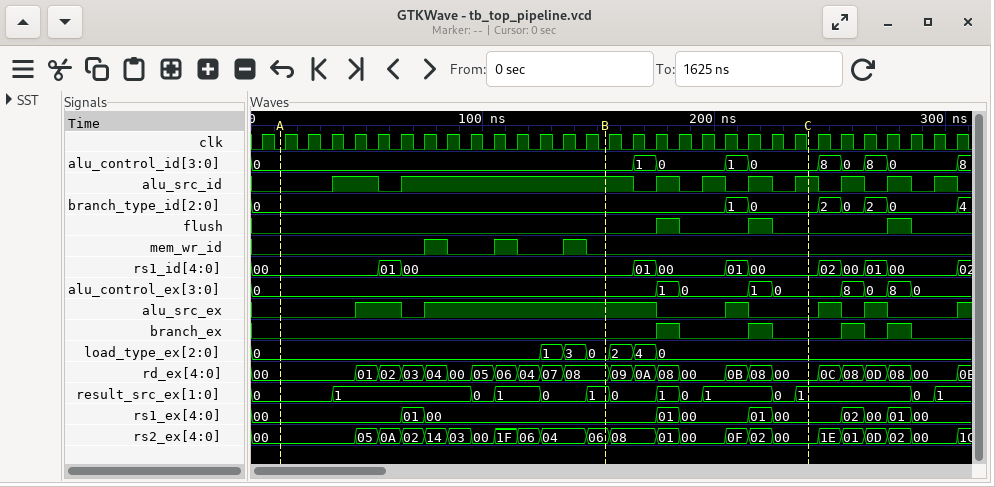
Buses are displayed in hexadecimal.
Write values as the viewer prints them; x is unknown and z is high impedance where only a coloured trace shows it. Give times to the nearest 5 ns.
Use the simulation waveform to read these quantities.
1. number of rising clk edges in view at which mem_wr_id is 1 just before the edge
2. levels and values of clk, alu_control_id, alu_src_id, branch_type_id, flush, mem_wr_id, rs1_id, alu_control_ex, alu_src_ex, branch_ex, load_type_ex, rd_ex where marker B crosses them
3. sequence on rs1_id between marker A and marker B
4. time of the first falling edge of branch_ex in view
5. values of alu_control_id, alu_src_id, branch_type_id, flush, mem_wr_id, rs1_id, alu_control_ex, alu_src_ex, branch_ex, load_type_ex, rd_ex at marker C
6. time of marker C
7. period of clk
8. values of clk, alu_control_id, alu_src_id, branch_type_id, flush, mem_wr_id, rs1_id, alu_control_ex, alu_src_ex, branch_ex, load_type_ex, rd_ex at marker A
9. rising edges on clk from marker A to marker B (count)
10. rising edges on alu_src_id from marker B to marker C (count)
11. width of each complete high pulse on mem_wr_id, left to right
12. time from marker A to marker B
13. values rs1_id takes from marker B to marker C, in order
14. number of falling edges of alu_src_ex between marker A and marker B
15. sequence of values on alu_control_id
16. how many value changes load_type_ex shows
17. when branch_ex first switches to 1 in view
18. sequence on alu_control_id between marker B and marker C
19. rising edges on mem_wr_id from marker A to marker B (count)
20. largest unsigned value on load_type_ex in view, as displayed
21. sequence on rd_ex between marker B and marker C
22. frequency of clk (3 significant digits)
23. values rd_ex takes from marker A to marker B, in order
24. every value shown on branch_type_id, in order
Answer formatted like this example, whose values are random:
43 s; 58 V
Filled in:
3; clk=0, alu_control_id=0, alu_src_id=1, branch_type_id=0, flush=0, mem_wr_id=0, rs1_id=00, alu_control_ex=0, alu_src_ex=1, branch_ex=0, load_type_ex=0, rd_ex=08; 00, 01, 00; 185 ns; alu_control_id=0, alu_src_id=1, branch_type_id=0, flush=0, mem_wr_id=0, rs1_id=00, alu_control_ex=0, alu_src_ex=0, branch_ex=0, load_type_ex=0, rd_ex=00; 240 ns; 10 ns; clk=0, alu_control_id=0, alu_src_id=0, branch_type_id=0, flush=0, mem_wr_id=0, rs1_id=00, alu_control_ex=0, alu_src_ex=0, branch_ex=0, load_type_ex=0, rd_ex=00; 14; 4; 10 ns, 10 ns, 10 ns; 140 ns; 00, 01, 00, 01, 00; 1; 0, 1, 0, 1, 0, 8, 0, 8, 0, 8; 6; 175 ns; 0, 1, 0, 1, 0; 3; 4; 08, 09, 0A, 08, 00, 0B, 08, 00; 100 MHz; 00, 01, 02, 03, 04, 00, 05, 06, 04, 07, 08; 0, 1, 0, 2, 0, 2, 0, 4
